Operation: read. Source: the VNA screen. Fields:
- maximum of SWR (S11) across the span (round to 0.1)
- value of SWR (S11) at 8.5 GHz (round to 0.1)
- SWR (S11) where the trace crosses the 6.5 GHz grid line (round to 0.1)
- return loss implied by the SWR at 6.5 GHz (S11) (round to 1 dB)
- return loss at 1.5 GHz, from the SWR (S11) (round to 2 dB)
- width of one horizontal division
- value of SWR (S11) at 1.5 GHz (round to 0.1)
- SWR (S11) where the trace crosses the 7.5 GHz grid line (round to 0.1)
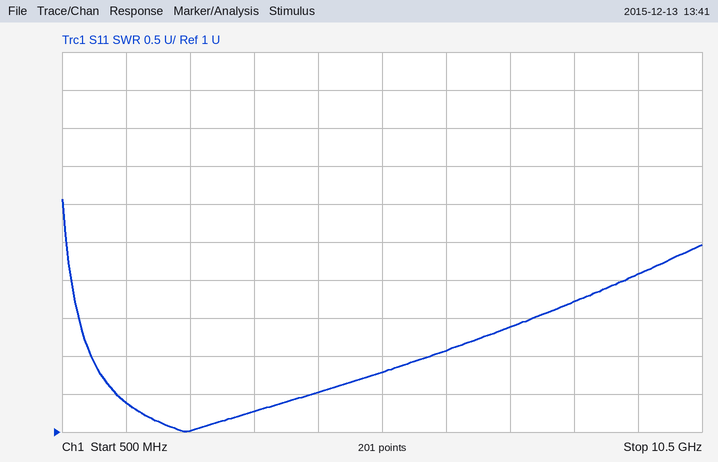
4.1
2.7
2.1
9 dB
16 dB
1 GHz
1.4
2.4
